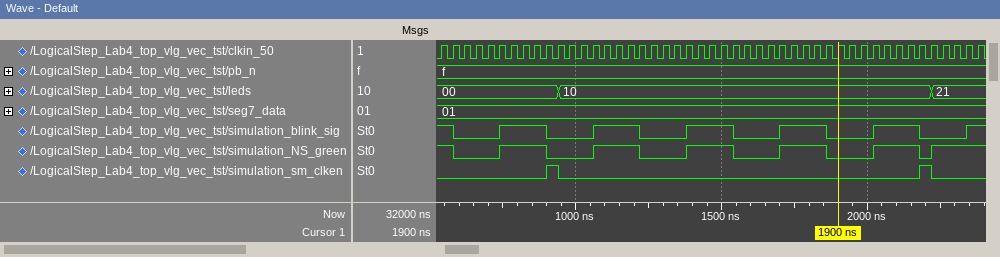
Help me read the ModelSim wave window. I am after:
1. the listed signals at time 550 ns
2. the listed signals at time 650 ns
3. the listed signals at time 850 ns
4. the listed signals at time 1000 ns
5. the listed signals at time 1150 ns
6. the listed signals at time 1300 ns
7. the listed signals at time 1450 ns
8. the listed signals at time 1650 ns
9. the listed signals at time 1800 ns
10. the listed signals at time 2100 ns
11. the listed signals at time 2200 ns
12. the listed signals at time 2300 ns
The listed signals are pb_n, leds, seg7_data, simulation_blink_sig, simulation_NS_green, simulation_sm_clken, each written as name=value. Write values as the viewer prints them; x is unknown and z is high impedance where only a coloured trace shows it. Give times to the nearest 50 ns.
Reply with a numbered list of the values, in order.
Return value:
1. pb_n=f, leds=00, seg7_data=01, simulation_blink_sig=1, simulation_NS_green=1, simulation_sm_clken=0
2. pb_n=f, leds=00, seg7_data=01, simulation_blink_sig=0, simulation_NS_green=0, simulation_sm_clken=0
3. pb_n=f, leds=00, seg7_data=01, simulation_blink_sig=1, simulation_NS_green=1, simulation_sm_clken=0
4. pb_n=f, leds=10, seg7_data=01, simulation_blink_sig=0, simulation_NS_green=0, simulation_sm_clken=0
5. pb_n=f, leds=10, seg7_data=01, simulation_blink_sig=1, simulation_NS_green=1, simulation_sm_clken=0
6. pb_n=f, leds=10, seg7_data=01, simulation_blink_sig=0, simulation_NS_green=0, simulation_sm_clken=0
7. pb_n=f, leds=10, seg7_data=01, simulation_blink_sig=1, simulation_NS_green=1, simulation_sm_clken=0
8. pb_n=f, leds=10, seg7_data=01, simulation_blink_sig=0, simulation_NS_green=0, simulation_sm_clken=0
9. pb_n=f, leds=10, seg7_data=01, simulation_blink_sig=1, simulation_NS_green=1, simulation_sm_clken=0
10. pb_n=f, leds=10, seg7_data=01, simulation_blink_sig=1, simulation_NS_green=1, simulation_sm_clken=0
11. pb_n=f, leds=10, seg7_data=01, simulation_blink_sig=0, simulation_NS_green=0, simulation_sm_clken=1
12. pb_n=f, leds=21, seg7_data=01, simulation_blink_sig=0, simulation_NS_green=1, simulation_sm_clken=0
